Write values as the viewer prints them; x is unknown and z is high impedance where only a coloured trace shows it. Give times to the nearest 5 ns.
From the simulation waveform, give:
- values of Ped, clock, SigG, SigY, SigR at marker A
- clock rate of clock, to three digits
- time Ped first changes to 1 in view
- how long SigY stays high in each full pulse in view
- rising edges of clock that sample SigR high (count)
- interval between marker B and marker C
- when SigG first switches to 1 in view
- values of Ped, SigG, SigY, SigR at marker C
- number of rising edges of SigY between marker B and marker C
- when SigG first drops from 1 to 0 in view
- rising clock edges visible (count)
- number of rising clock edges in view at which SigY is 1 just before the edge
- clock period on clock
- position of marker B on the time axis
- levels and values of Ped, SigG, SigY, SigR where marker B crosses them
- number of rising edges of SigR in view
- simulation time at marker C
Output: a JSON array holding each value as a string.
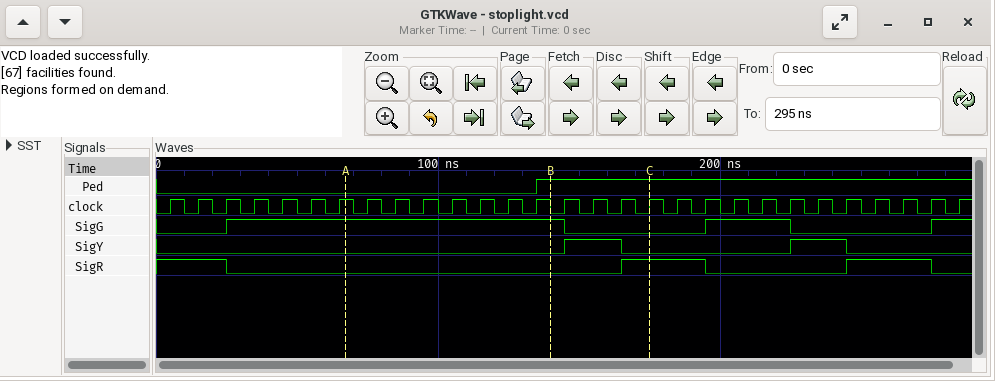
["Ped=0, clock=1, SigG=1, SigY=0, SigR=0", "100 MHz", "135 ns", "20 ns, 20 ns", "9", "35 ns", "25 ns", "Ped=1, SigG=0, SigY=0, SigR=1", "1", "145 ns", "29", "4", "10 ns", "140 ns", "Ped=1, SigG=1, SigY=0, SigR=0", "2", "175 ns"]
